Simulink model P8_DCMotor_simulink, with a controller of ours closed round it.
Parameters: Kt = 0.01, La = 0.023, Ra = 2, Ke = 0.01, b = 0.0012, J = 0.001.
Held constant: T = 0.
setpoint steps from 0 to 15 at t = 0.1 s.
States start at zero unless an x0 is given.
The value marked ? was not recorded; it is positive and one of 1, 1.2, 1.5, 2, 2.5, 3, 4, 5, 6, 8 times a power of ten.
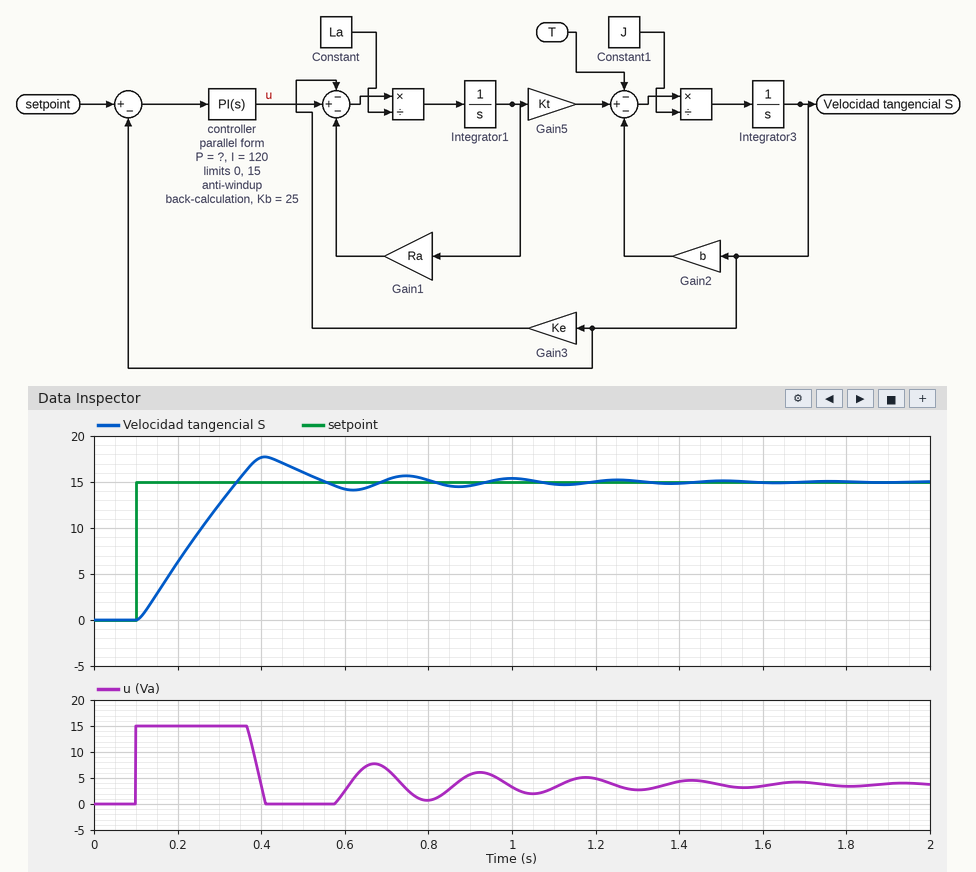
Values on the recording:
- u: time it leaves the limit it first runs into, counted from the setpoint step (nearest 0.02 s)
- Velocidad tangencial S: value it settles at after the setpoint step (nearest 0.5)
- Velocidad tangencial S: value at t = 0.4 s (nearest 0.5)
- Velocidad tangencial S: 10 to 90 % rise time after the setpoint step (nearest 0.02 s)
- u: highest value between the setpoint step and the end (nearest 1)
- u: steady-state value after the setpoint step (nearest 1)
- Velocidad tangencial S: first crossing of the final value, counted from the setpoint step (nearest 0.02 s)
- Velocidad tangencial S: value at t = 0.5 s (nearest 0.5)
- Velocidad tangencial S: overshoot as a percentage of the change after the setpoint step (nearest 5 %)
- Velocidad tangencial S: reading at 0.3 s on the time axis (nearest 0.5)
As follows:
0.26 s
15.0
17.5
0.18 s
15
4
0.24 s
16.0
20 %
12.5
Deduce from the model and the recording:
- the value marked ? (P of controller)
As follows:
2
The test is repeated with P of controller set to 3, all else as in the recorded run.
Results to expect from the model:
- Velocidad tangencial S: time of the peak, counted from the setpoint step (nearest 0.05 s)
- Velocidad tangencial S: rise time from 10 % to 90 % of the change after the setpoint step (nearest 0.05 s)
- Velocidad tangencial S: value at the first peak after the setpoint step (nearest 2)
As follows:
0.30 s
0.20 s
18
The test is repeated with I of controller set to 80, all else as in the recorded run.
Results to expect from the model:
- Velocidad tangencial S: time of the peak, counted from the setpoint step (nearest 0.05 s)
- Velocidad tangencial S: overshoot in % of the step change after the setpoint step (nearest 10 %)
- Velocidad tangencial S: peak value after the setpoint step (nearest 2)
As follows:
0.30 s
20 %
18
